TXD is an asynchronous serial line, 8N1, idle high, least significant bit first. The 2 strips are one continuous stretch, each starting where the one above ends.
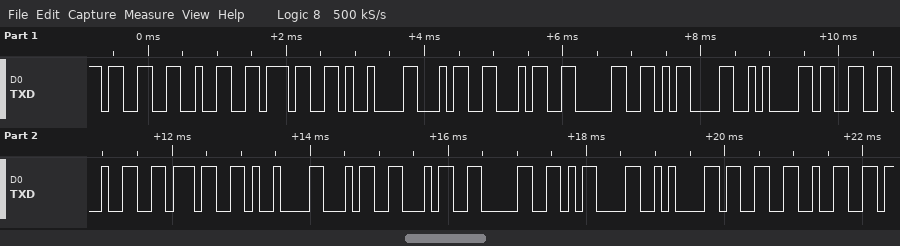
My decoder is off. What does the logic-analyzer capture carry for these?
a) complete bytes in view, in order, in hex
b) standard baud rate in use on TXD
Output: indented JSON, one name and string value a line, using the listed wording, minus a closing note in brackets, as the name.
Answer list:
{
  "complete bytes in view, in order, in hex": "0x33 0x32 0x37 0x09 0x34 0x34 0x30 0x0D 0x0A 0x33 0x32 0x37 0x09 0x34 0x34 0x30 0x0D 0x0A 0x33 0x32",
  "standard baud rate in use on TXD": "9600 baud"
}
